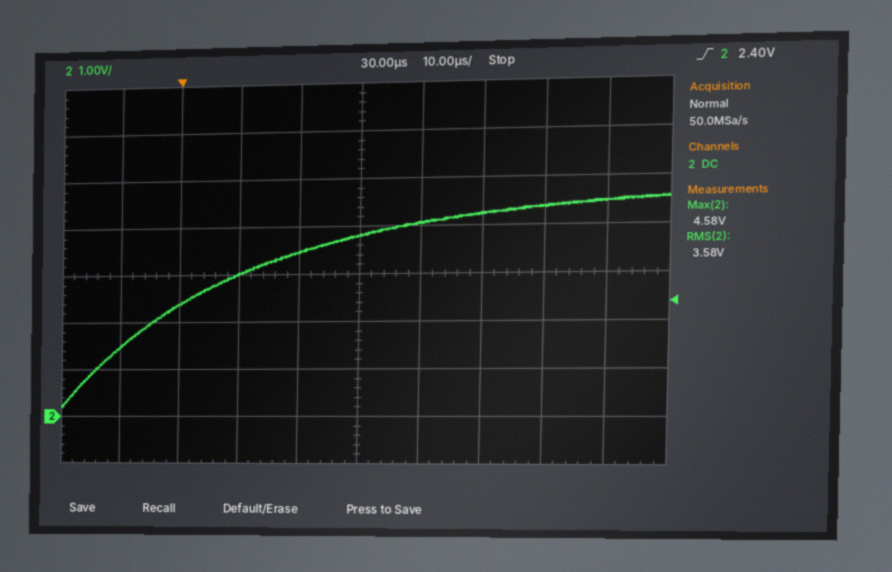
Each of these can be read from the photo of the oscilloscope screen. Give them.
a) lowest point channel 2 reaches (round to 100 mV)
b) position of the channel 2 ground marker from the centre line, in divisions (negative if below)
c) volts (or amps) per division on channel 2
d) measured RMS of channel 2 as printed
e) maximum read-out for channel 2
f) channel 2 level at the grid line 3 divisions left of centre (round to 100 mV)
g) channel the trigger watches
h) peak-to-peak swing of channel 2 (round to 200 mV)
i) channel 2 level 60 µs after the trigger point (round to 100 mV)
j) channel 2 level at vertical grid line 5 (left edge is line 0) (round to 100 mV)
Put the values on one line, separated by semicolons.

200 mV; -3.0 div; 1 V; 3.58 V; 4.58 V; 2.4 V; channel 2; 4.4 V; 4.4 V; 3.8 V
